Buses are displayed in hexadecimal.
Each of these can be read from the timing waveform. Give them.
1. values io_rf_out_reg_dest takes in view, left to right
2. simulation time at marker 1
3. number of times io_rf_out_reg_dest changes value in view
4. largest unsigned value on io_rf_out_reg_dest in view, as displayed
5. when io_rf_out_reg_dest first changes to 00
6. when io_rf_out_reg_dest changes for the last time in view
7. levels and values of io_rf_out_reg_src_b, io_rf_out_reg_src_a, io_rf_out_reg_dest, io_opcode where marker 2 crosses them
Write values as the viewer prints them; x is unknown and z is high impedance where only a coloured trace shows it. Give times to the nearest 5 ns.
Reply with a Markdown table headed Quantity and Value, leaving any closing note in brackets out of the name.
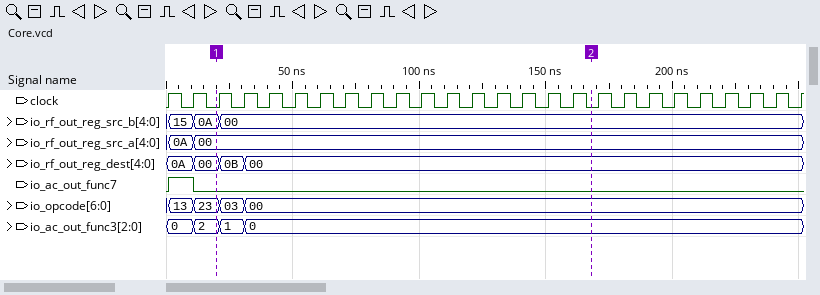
| Quantity | Value |
|---|---|
| values io_rf_out_reg_dest takes in view, left to right | 0A, 00, 0B, 00 |
| simulation time at marker 1 | 20 ns |
| number of times io_rf_out_reg_dest changes value in view | 3 |
| largest unsigned value on io_rf_out_reg_dest in view, as displayed | 0B |
| when io_rf_out_reg_dest first changes to 00 | 10 ns |
| when io_rf_out_reg_dest changes for the last time in view | 30 ns |
| levels and values of io_rf_out_reg_src_b, io_rf_out_reg_src_a, io_rf_out_reg_dest, io_opcode where marker 2 crosses them | io_rf_out_reg_src_b=00, io_rf_out_reg_src_a=00, io_rf_out_reg_dest=00, io_opcode=00 |
